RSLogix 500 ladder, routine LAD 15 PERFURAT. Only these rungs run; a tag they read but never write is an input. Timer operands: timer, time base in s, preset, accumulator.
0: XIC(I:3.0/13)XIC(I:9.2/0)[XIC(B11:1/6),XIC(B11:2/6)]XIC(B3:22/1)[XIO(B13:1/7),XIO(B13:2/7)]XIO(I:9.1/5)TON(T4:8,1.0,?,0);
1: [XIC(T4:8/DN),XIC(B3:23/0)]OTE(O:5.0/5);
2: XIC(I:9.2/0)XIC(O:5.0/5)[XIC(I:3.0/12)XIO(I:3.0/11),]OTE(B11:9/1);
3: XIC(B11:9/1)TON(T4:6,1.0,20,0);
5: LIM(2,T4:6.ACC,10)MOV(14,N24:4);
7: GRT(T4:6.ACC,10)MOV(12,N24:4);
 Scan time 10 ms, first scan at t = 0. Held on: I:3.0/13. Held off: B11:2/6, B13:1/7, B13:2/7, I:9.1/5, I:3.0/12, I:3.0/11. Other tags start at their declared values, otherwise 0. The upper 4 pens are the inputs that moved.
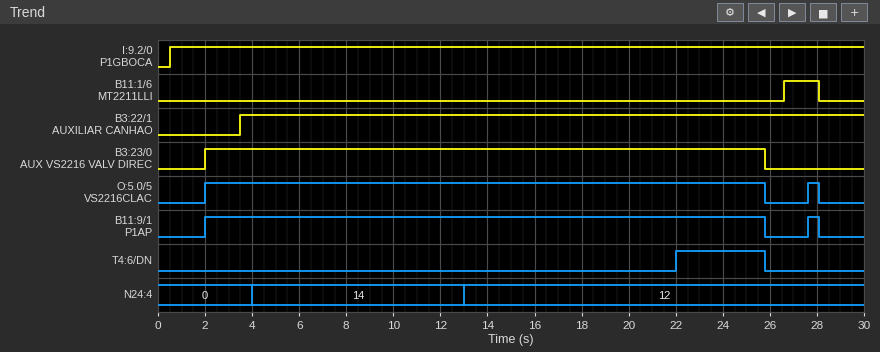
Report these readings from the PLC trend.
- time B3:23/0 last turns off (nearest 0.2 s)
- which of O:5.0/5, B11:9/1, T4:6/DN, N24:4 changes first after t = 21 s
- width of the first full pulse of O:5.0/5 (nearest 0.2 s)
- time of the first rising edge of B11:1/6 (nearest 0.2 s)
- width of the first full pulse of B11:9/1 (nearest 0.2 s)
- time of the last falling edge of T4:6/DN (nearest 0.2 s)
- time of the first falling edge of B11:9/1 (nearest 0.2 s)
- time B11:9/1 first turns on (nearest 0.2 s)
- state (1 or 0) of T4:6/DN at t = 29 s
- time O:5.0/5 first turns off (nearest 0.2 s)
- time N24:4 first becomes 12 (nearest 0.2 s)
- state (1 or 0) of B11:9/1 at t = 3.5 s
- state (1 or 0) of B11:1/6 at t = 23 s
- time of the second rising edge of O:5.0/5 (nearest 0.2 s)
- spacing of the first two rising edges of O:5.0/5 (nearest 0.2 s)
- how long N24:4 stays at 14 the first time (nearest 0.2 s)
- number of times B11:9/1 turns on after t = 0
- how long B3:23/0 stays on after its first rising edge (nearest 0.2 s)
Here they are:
25.8 s
T4:6/DN
23.8 s
26.6 s
23.8 s
25.8 s
25.8 s
2.0 s
0
25.8 s
13.0 s
1
0
27.6 s
25.6 s
9.0 s
2
23.8 s
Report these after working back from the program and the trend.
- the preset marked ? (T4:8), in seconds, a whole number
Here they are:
1 s
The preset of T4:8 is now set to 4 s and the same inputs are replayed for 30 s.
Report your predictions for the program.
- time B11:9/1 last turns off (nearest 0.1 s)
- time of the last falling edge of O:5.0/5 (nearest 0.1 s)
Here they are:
25.8 s
25.8 s
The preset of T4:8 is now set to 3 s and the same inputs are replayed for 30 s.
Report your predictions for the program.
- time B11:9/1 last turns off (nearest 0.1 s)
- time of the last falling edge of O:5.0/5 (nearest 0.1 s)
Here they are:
25.8 s
25.8 s
